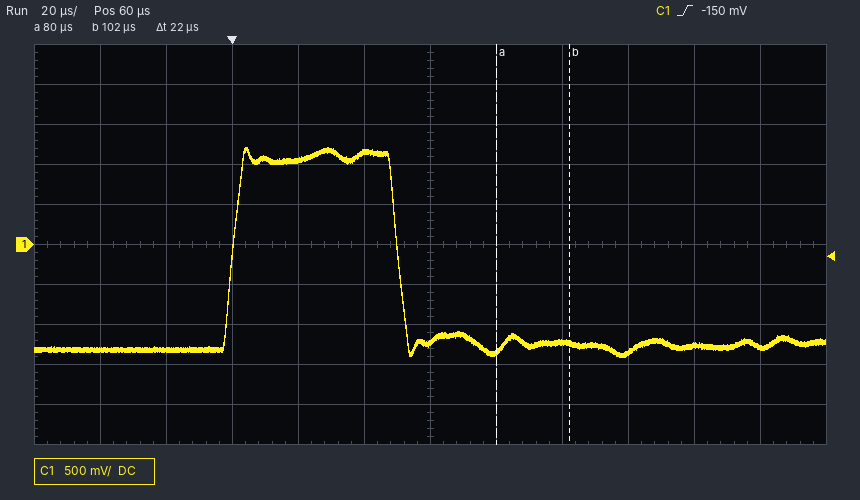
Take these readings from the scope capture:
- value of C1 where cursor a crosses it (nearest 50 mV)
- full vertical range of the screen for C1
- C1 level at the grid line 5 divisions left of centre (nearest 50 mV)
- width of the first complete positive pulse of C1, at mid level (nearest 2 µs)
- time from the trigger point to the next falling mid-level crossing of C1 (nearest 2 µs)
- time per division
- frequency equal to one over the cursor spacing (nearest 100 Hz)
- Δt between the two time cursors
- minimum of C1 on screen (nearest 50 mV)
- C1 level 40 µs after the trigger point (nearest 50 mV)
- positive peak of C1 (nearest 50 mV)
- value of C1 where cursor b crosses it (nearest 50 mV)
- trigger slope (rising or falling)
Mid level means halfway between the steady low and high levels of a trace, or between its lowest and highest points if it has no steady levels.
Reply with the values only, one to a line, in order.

-1.35 V
5 V
-1.30 V
50 µs
50 µs
20 µs
45.5 kHz
22 µs
-1.40 V
1.15 V
1.20 V
-1.25 V
rising
